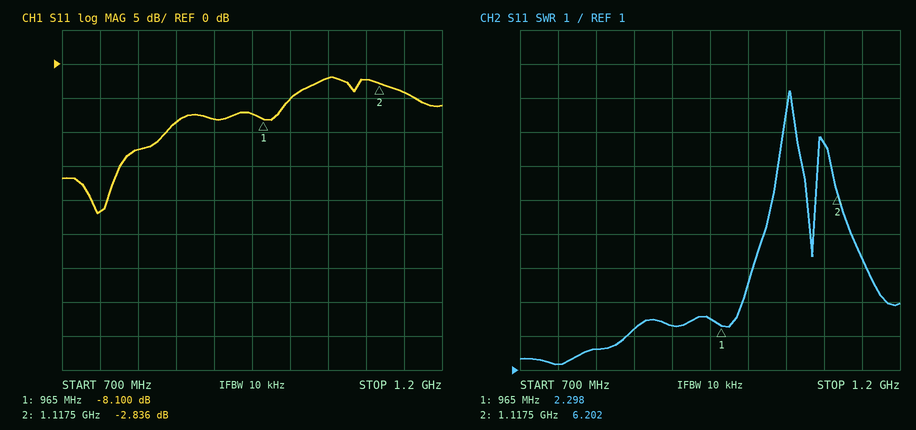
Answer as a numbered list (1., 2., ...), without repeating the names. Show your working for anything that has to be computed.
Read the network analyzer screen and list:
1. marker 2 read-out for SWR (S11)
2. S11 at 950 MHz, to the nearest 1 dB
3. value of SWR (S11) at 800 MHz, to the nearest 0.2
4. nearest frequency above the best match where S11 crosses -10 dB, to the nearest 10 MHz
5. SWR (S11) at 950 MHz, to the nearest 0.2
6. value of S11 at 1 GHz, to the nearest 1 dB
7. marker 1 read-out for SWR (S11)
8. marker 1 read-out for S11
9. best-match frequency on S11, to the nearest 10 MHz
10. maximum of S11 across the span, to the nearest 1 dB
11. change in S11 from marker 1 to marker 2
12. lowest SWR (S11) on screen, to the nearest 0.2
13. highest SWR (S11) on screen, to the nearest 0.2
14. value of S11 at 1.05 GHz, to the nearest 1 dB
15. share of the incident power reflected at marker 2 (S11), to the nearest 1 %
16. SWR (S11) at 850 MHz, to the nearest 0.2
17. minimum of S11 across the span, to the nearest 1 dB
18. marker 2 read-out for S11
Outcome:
1. 6.202
2. -7 dB
3. 1.6
4. 840 MHz
5. 2.6
6. -5 dB
7. 2.298
8. -8.100 dB
9. 750 MHz
10. -2 dB
11. -2.836 − (-8.1) = 5.264 dB
12. 1.2
13. 9.2
14. -2 dB
15. 10^(-2.836/10) ≈ 52 %
16. 2.2
17. -22 dB
18. -2.836 dB
